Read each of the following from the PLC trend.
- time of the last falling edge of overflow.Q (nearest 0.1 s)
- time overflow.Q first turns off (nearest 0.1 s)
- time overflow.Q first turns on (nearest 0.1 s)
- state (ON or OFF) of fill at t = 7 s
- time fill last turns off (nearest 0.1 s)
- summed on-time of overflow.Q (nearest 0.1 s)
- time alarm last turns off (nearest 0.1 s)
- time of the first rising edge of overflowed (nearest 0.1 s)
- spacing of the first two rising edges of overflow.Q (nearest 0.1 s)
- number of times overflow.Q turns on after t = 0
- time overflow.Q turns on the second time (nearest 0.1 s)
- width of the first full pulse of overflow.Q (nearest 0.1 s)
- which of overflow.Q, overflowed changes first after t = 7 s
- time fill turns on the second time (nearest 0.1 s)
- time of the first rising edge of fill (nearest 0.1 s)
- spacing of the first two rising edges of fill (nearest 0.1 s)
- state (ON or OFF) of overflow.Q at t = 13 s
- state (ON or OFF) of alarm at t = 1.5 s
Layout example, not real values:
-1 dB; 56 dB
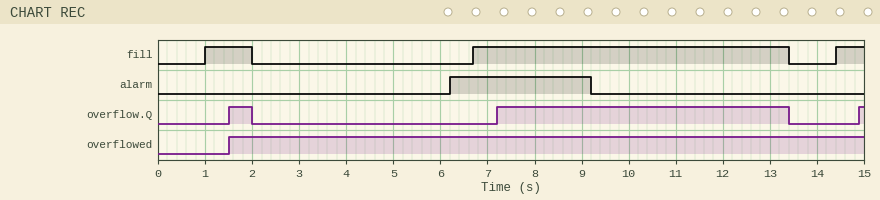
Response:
13.4 s; 2.0 s; 1.5 s; ON; 13.4 s; 6.8 s; 9.2 s; 1.5 s; 5.7 s; 3; 7.2 s; 0.5 s; overflow.Q; 6.7 s; 1.0 s; 5.7 s; ON; OFF
